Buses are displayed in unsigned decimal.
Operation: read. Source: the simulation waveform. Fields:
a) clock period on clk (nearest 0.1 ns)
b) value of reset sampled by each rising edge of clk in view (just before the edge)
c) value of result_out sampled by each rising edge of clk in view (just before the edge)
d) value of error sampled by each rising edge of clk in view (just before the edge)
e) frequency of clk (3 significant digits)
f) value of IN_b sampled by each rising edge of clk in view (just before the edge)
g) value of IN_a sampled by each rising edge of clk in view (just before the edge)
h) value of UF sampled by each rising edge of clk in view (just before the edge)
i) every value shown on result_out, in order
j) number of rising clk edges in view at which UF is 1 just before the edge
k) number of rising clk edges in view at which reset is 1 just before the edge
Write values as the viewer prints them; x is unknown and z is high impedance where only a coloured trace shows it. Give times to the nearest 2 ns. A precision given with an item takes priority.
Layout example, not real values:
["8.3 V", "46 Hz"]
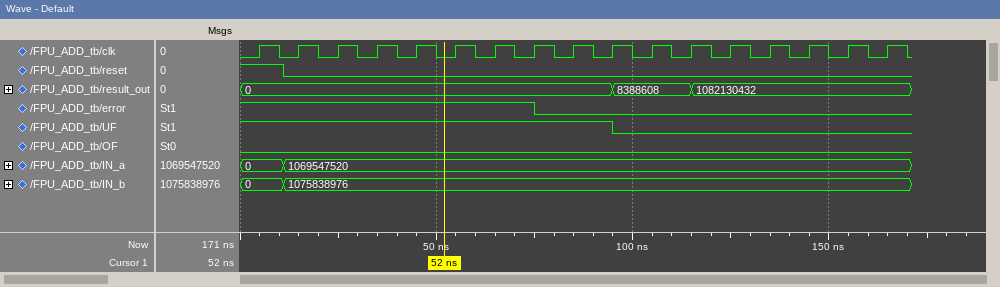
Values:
["10 ns", "1 0 0 0 0 0 0 0 0 0 0 0 0 0 0 0 0", "0, 0, 0, 0, 0, 0, 0, 0, 0, 0, 8388608, 8388608, 1082130432, 1082130432, 1082130432, 1082130432, 1082130432", "1 1 1 1 1 1 1 1 0 0 0 0 0 0 0 0 0", "100 MHz", "0, 1075838976, 1075838976, 1075838976, 1075838976, 1075838976, 1075838976, 1075838976, 1075838976, 1075838976, 1075838976, 1075838976, 1075838976, 1075838976, 1075838976, 1075838976, 1075838976", "0, 1069547520, 1069547520, 1069547520, 1069547520, 1069547520, 1069547520, 1069547520, 1069547520, 1069547520, 1069547520, 1069547520, 1069547520, 1069547520, 1069547520, 1069547520, 1069547520", "1 1 1 1 1 1 1 1 1 1 0 0 0 0 0 0 0", "0, 8388608, 1082130432", "10", "1"]
